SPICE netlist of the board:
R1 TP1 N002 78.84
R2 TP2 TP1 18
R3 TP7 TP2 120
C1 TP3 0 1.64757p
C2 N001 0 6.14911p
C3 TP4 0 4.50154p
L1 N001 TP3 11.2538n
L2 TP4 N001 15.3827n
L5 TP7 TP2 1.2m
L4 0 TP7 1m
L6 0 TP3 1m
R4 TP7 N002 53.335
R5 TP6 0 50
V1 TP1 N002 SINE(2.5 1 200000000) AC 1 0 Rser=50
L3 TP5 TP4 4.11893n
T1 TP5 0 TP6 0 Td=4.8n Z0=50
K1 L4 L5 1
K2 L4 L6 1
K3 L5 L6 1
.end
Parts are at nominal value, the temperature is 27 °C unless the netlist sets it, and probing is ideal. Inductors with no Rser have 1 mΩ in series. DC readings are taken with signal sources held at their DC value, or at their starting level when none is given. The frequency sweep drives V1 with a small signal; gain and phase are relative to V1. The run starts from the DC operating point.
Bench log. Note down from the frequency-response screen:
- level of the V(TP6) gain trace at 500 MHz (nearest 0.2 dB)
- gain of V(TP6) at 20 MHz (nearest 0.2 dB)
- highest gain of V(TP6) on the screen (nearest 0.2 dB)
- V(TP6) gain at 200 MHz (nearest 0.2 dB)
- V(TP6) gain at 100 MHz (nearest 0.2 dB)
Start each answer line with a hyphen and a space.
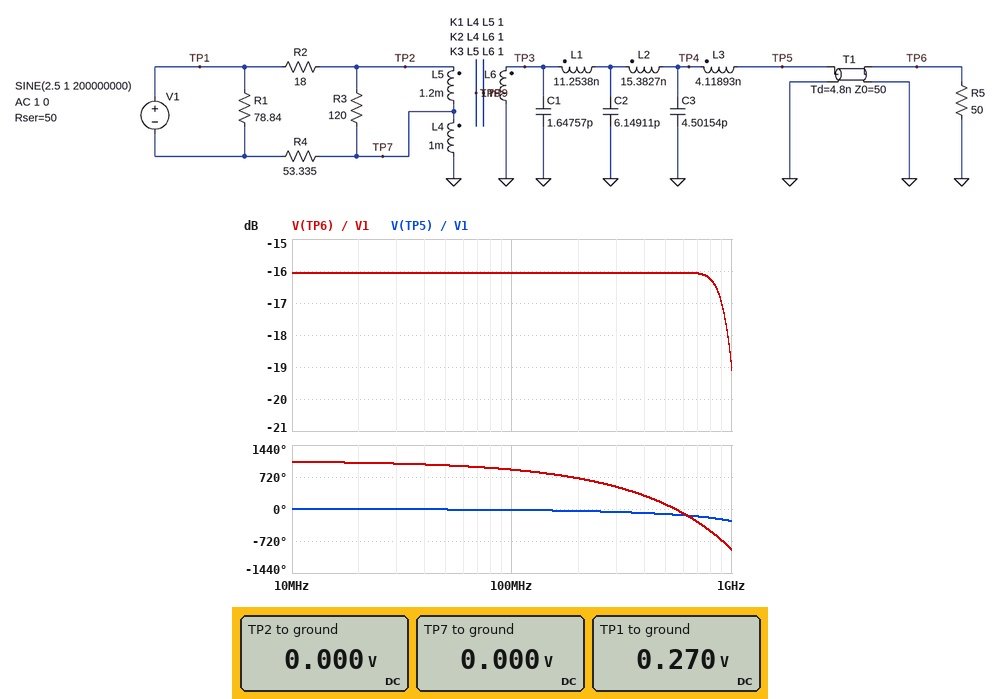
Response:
- -16.0 dB
- -16.0 dB
- -16.0 dB
- -16.0 dB
- -16.0 dB
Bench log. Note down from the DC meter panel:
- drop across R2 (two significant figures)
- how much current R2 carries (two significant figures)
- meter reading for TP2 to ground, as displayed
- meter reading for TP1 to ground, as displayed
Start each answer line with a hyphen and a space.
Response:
- 270 mV
- 15 mA
- 0.000 V
- 0.270 V
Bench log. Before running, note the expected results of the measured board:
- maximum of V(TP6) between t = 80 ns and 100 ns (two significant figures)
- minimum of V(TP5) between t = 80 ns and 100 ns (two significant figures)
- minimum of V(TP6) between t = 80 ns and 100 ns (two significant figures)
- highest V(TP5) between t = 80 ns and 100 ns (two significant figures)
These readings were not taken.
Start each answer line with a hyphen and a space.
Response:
- 160 mV
- -160 mV
- -160 mV
- 160 mV
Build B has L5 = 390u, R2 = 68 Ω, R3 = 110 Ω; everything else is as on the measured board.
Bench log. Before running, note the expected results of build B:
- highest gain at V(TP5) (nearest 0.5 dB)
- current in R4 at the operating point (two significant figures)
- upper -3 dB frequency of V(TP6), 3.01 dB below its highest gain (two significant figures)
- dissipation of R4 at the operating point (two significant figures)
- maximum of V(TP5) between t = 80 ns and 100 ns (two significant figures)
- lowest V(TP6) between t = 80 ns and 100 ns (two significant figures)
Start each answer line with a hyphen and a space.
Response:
- -20.5 dB
- 10 mA
- 950 MHz
- 5.4 mW
- 96 mV
- -96 mV
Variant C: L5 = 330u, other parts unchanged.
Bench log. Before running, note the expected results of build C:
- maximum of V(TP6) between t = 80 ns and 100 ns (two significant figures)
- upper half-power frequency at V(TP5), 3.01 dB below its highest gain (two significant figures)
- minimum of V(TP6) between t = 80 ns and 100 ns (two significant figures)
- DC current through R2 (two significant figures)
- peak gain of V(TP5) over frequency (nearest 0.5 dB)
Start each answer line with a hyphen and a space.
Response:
- 130 mV
- 950 MHz
- -130 mV
- 15 mA
- -17.5 dB
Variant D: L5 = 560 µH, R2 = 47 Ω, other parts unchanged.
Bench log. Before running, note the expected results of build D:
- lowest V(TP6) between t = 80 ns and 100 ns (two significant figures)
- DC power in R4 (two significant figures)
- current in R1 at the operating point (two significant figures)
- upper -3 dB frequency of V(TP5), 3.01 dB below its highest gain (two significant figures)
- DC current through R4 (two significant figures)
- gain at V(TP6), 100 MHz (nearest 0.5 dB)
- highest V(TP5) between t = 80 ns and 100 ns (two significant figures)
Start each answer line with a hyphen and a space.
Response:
- -120 mV
- 7.3 mW
- 15 mA
- 980 MHz
- 12 mA
- -18.5 dB
- 120 mV
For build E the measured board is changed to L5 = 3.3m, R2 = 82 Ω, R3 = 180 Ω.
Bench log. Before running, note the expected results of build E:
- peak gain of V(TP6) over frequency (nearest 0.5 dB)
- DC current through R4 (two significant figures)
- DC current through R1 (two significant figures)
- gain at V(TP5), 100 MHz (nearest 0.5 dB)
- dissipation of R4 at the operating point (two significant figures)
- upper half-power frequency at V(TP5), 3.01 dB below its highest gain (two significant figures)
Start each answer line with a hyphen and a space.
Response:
- -18.5 dB
- 9.2 mA
- 16 mA
- -19.0 dB
- 4.5 mW
- 980 MHz
